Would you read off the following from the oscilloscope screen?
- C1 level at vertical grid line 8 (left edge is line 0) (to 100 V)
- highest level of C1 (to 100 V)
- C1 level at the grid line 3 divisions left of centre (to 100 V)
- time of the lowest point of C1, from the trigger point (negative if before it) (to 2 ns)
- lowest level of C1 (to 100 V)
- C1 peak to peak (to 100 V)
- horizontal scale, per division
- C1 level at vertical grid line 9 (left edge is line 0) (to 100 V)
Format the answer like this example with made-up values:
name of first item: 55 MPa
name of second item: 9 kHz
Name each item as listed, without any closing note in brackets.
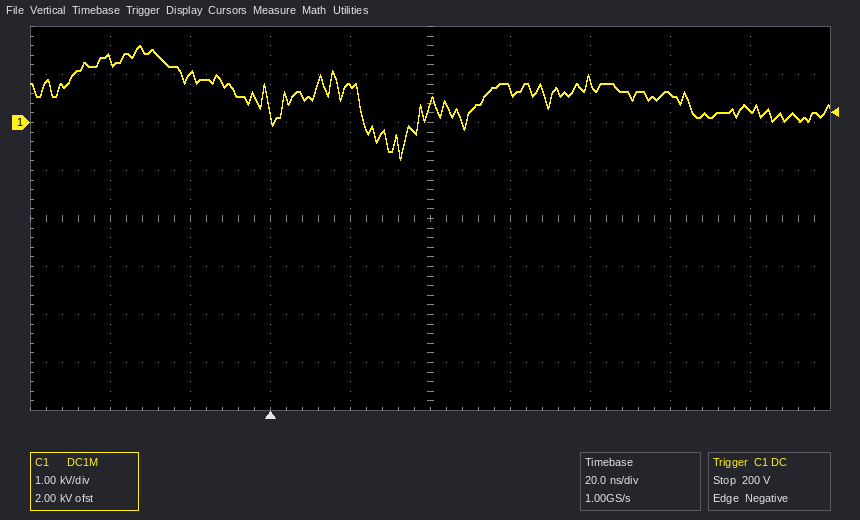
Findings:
C1 level at vertical grid line 8 (left edge is line 0): 600 V
highest level of C1: 1.6 kV
C1 level at the grid line 3 divisions left of centre: 1.0 kV
time of the lowest point of C1, from the trigger point (negative if before it): +32 ns
lowest level of C1: -800 V
C1 peak to peak: 2.4 kV
horizontal scale, per division: 20 ns
C1 level at vertical grid line 9 (left edge is line 0): 300 V
